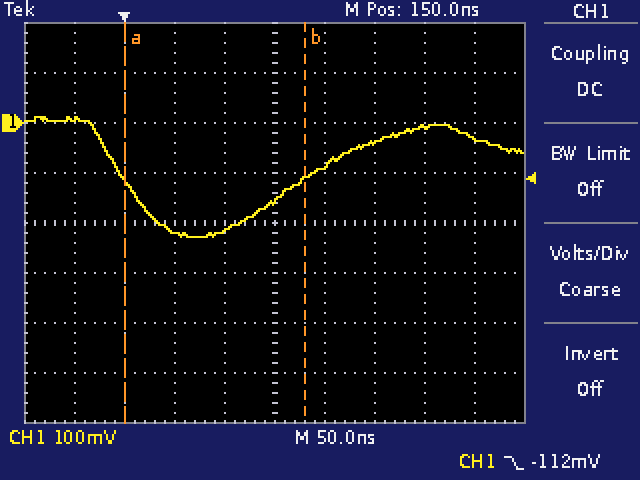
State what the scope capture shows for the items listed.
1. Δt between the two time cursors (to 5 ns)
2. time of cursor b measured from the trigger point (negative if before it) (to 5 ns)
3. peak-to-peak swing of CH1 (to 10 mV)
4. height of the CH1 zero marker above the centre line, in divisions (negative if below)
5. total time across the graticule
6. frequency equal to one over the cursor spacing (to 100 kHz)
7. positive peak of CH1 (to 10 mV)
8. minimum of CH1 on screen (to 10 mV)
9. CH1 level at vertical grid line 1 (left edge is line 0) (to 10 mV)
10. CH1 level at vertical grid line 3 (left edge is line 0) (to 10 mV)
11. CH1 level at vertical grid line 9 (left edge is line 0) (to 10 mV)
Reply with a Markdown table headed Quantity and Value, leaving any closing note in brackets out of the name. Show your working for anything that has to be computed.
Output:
| Quantity | Value |
|---|---|
| Δt between the two time cursors | 180 ns |
| time of cursor b measured from the trigger point (negative if before it) | +180 ns |
| peak-to-peak swing of CH1 | 10 mV − (-230 mV) = 240 mV |
| height of the CH1 zero marker above the centre line, in divisions | +2.0 div |
| total time across the graticule | 500 ns |
| frequency equal to one over the cursor spacing | 1 / 180 ns ≈ 5.6 MHz |
| positive peak of CH1 | 10 mV |
| minimum of CH1 on screen | -230 mV |
| CH1 level at vertical grid line 1 (left edge is line 0) | 10 mV |
| CH1 level at vertical grid line 3 (left edge is line 0) | -220 mV |
| CH1 level at vertical grid line 9 (left edge is line 0) | -30 mV |
